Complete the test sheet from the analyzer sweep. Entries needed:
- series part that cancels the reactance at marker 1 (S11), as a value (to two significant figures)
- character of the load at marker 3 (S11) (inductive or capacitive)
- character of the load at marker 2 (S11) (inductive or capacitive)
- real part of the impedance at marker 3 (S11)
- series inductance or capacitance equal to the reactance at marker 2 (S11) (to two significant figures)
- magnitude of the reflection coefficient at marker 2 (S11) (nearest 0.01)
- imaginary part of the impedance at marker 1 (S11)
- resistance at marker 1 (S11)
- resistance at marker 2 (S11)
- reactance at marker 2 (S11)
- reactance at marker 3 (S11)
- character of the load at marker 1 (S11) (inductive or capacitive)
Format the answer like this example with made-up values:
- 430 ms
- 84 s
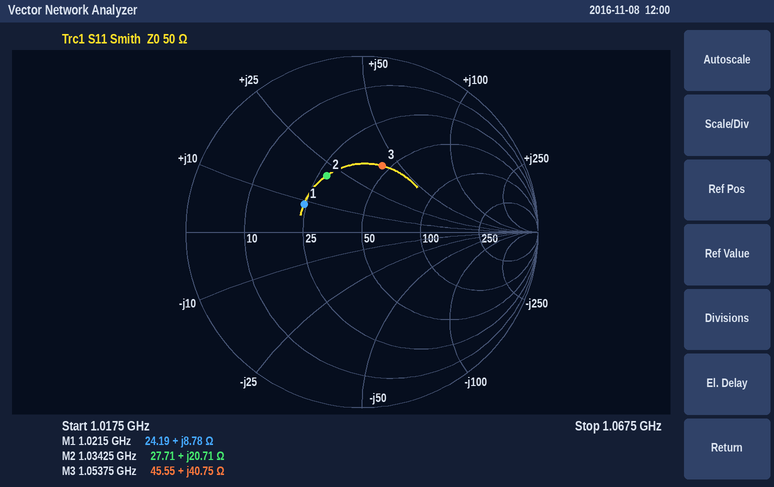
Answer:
- 18 pF
- inductive
- inductive
- 45.55 Ω
- 3.2 nH
- 0.38
- +8.78 Ω
- 24.19 Ω
- 27.71 Ω
- +20.71 Ω
- +40.75 Ω
- inductive
